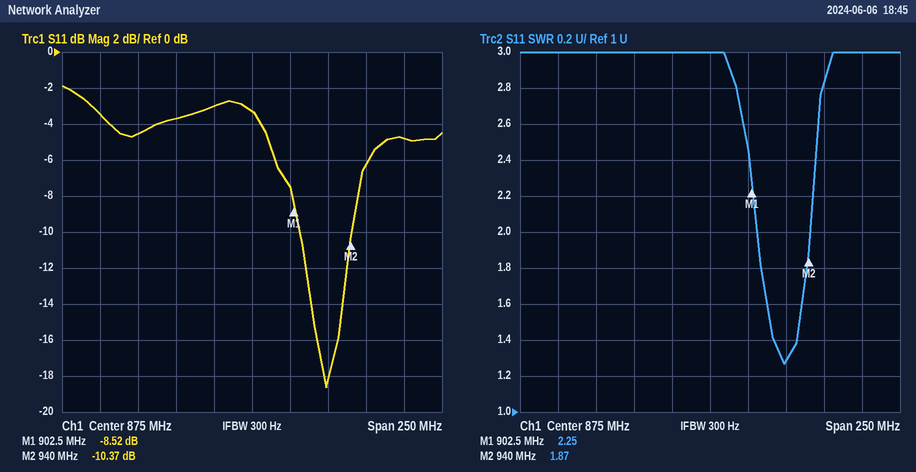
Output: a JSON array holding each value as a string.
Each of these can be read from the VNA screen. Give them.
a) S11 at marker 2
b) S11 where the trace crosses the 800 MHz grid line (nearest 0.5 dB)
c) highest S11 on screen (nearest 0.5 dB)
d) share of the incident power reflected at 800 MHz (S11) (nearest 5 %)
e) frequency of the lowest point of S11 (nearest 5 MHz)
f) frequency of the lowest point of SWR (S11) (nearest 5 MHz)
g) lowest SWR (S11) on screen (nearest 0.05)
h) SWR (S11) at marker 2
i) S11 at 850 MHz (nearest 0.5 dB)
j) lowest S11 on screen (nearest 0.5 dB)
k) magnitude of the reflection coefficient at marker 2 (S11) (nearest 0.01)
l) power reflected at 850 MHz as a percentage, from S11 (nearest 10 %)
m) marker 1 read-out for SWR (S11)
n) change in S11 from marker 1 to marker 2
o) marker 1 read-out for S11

["-10.37 dB", "-4.5 dB", "-2.0 dB", "35 %", "925 MHz", "925 MHz", "1.25", "1.87", "-3.0 dB", "-18.5 dB", "0.30", "50 %", "2.25", "-1.85 dB", "-8.52 dB"]
